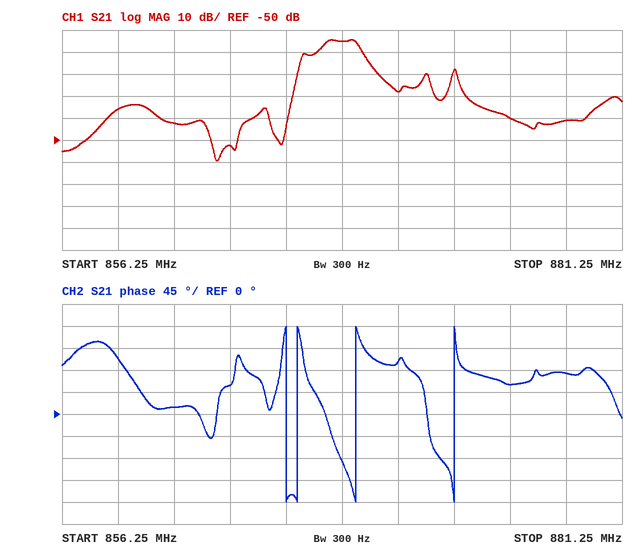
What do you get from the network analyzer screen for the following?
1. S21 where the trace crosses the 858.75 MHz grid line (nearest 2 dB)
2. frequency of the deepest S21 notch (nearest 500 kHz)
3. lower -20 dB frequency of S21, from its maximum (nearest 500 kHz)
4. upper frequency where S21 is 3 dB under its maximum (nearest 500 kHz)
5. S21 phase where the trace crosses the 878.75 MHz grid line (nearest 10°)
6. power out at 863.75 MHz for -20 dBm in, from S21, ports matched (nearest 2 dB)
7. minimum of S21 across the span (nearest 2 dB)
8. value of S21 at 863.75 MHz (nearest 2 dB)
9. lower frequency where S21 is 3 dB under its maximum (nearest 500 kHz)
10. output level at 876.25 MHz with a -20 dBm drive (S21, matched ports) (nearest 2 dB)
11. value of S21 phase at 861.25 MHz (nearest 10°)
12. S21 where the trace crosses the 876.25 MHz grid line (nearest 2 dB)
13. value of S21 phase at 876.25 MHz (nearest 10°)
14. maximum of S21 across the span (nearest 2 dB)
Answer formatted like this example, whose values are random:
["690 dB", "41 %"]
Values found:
["-36 dB", "863.0 MHz", "866.5 MHz", "869.5 MHz", "80°", "-72 dBm", "-60 dB", "-52 dB", "868.0 MHz", "-60 dBm", "10°", "-40 dB", "60°", "-4 dB"]
